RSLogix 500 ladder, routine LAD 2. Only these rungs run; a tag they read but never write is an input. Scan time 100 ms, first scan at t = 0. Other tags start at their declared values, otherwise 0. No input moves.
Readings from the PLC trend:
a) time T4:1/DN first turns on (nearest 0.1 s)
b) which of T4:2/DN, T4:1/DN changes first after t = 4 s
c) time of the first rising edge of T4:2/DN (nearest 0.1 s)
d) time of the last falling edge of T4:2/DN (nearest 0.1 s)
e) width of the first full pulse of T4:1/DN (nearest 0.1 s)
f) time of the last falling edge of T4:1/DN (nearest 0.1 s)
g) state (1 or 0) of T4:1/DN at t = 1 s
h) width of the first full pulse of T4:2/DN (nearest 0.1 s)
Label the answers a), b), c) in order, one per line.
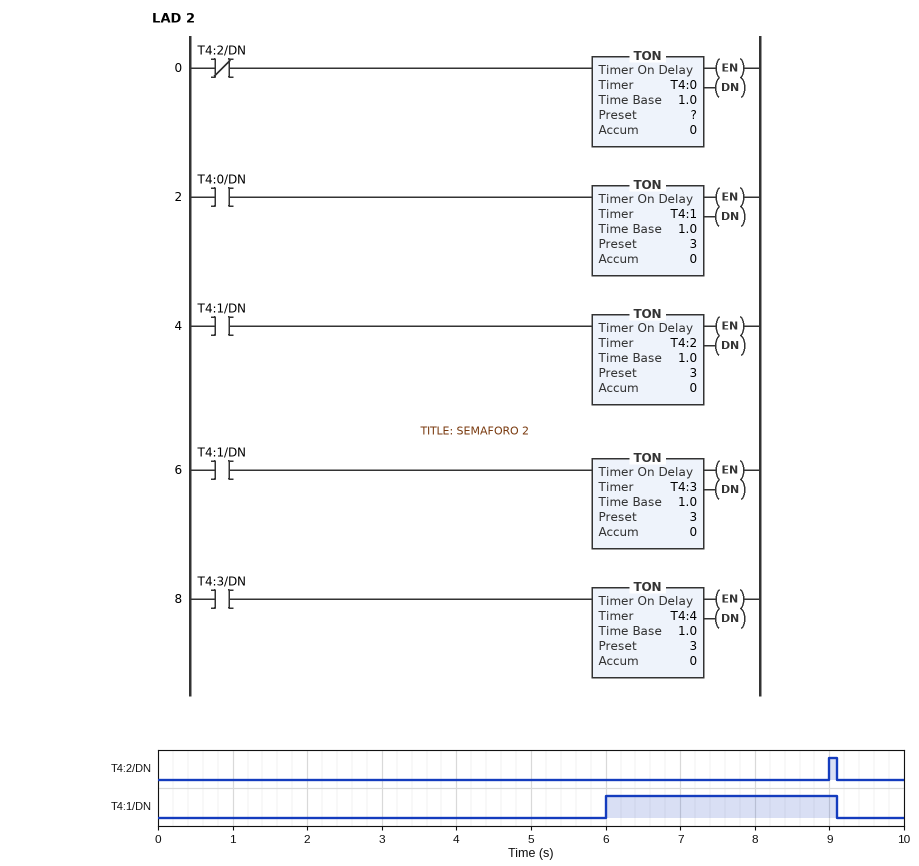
a) 6.0 s
b) T4:1/DN
c) 9.0 s
d) 9.1 s
e) 3.1 s
f) 9.1 s
g) 0
h) 0.1 s
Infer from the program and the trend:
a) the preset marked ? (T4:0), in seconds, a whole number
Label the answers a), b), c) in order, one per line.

a) 3 s
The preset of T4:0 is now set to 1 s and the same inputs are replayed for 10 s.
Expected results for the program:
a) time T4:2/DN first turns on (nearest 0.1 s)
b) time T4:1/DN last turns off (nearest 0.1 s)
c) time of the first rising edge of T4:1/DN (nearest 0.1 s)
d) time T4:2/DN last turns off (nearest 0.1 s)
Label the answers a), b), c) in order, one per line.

a) 7.0 s
b) 7.1 s
c) 4.0 s
d) 7.1 s
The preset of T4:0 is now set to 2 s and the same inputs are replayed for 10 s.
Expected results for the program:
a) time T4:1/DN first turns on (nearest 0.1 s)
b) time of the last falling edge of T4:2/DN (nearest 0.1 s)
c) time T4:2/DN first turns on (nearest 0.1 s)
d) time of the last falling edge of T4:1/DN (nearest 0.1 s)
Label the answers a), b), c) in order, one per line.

a) 5.0 s
b) 8.1 s
c) 8.0 s
d) 8.1 s
